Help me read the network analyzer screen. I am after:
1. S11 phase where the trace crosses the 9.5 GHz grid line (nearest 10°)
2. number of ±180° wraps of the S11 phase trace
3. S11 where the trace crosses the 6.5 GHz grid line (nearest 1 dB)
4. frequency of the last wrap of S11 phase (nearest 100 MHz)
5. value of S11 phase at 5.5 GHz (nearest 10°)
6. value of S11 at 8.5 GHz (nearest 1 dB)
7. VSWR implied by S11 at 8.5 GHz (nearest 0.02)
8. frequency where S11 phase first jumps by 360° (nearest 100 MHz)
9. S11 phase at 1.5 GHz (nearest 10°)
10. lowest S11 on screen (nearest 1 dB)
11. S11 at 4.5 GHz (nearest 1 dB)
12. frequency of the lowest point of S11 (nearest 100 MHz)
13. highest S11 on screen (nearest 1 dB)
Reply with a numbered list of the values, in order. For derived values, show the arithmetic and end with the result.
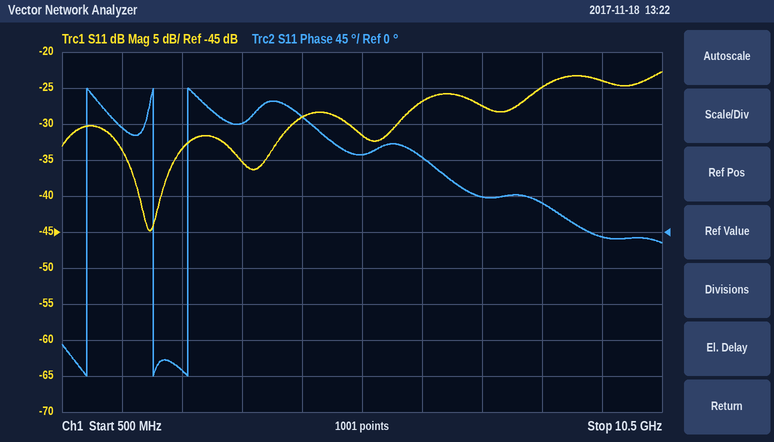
1. -10°
2. 3
3. -27 dB
4. 2.6 GHz
5. 100°
6. -25 dB
7. |Γ| = 10^(-25/20) = 0.0562; VSWR = (1 + 0.0562)/(1 − 0.0562) ≈ 1.12
8. 900 MHz
9. 130°
10. -45 dB
11. -29 dB
12. 2.0 GHz
13. -23 dB
